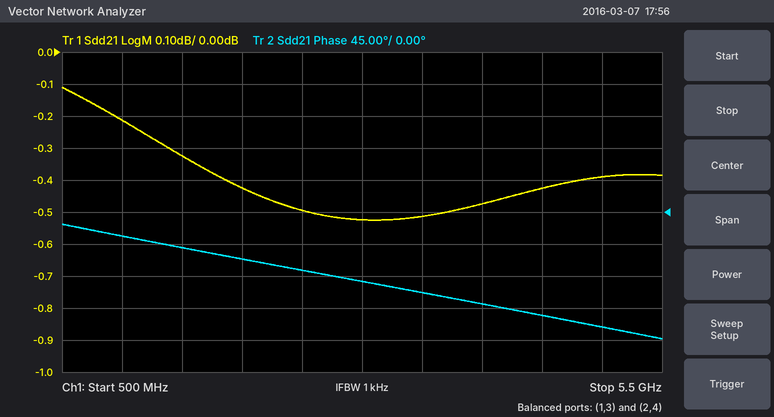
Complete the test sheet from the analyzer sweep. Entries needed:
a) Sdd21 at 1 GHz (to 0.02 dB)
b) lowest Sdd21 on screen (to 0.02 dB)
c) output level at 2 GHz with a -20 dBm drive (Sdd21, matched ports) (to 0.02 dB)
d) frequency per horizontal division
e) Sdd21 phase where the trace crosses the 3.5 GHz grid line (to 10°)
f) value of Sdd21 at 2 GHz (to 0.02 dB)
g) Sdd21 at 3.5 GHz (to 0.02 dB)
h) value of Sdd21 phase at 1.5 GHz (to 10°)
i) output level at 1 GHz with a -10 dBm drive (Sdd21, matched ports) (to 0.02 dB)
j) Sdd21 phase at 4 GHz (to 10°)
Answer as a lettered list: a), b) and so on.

a) -0.22 dB
b) -0.52 dB
c) -20.42 dBm
d) 500 MHz
e) -110°
f) -0.42 dB
g) -0.52 dB
h) -50°
i) -10.22 dBm
j) -130°
